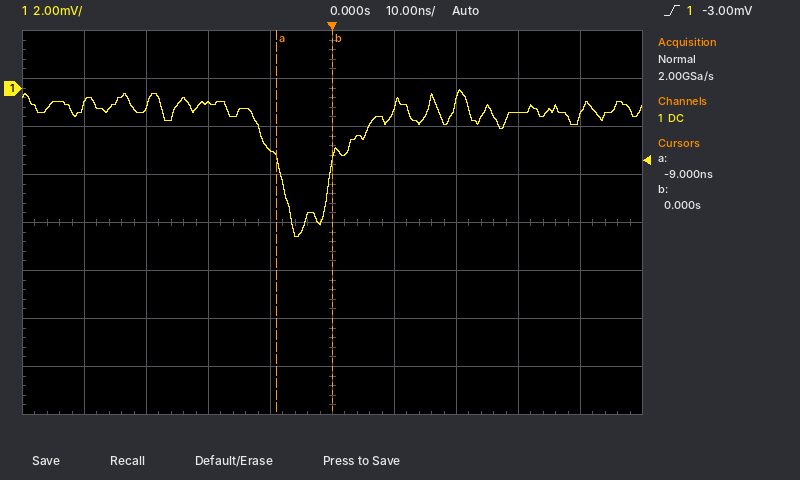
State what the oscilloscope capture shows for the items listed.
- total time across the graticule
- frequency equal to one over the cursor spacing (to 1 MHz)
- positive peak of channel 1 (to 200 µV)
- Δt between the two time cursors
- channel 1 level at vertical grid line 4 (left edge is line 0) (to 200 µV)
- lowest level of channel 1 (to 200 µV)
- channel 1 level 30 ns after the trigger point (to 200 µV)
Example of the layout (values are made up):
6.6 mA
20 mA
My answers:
100 ns
111 MHz
0.0 mV
9 ns
-2.6 mV
-6.2 mV
-1.0 mV
